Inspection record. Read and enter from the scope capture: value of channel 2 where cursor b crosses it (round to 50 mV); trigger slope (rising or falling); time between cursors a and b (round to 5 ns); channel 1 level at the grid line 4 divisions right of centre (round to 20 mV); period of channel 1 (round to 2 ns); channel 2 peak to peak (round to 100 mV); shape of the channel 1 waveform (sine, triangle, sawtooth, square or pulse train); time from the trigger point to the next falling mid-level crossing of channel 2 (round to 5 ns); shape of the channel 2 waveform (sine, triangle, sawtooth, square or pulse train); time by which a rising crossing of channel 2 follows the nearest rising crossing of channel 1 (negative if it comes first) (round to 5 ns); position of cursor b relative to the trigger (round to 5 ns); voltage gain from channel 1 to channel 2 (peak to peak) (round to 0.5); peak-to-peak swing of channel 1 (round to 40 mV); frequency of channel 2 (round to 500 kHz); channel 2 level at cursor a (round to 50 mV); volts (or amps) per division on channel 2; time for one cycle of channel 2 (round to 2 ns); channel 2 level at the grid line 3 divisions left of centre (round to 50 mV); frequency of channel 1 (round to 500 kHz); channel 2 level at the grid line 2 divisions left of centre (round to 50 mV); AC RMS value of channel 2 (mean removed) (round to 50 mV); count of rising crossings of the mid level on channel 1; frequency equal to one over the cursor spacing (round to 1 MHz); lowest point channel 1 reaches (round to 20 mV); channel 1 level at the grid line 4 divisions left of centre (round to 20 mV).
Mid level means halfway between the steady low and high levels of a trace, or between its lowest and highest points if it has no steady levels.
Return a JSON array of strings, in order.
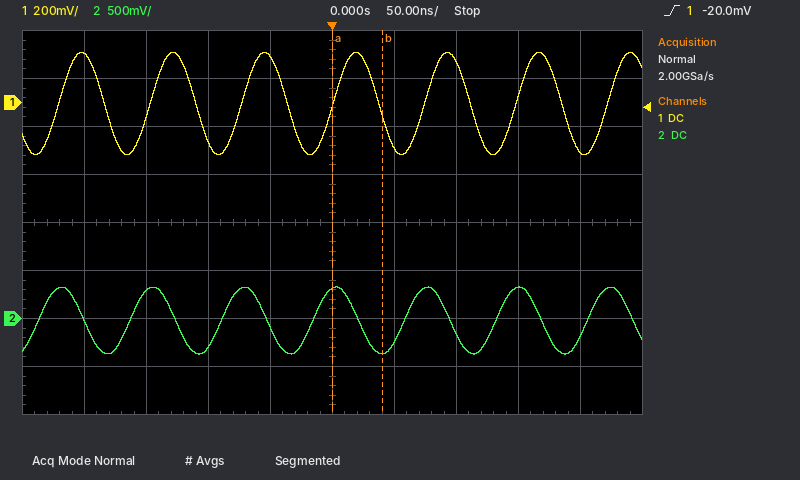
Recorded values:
["-350 mV", "rising", "40 ns", "-200 mV", "74 ns", "700 mV", "sine", "20 ns", "sine", "-15 ns", "+40 ns", "1.5", "440 mV", "13.5 MHz", "300 mV", "500 mV", "74 ns", "300 mV", "13.5 MHz", "-300 mV", "250 mV", "7", "25 MHz", "-220 mV", "200 mV"]
